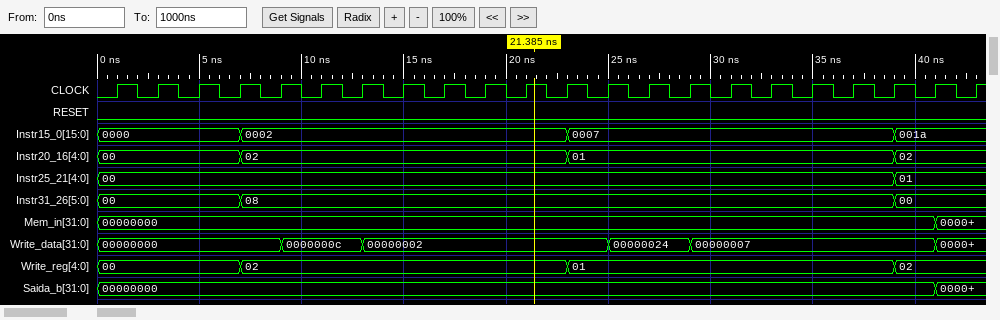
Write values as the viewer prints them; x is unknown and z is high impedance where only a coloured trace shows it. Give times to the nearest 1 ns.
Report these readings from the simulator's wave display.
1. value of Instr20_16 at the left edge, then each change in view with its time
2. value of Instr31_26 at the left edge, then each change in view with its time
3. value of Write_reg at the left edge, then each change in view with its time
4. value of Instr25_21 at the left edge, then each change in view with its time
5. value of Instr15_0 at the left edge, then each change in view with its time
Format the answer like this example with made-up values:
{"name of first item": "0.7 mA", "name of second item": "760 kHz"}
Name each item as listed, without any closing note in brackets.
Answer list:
{"value of Instr20_16 at the left edge, then each change in view with its time": "00, 02 at 7 ns, 01 at 23 ns, 02 at 39 ns", "value of Instr31_26 at the left edge, then each change in view with its time": "00, 08 at 7 ns, 00 at 39 ns", "value of Write_reg at the left edge, then each change in view with its time": "00, 02 at 7 ns, 01 at 23 ns, 02 at 39 ns", "value of Instr25_21 at the left edge, then each change in view with its time": "00, 01 at 39 ns", "value of Instr15_0 at the left edge, then each change in view with its time": "0000, 0002 at 7 ns, 0007 at 23 ns, 001a at 39 ns"}
